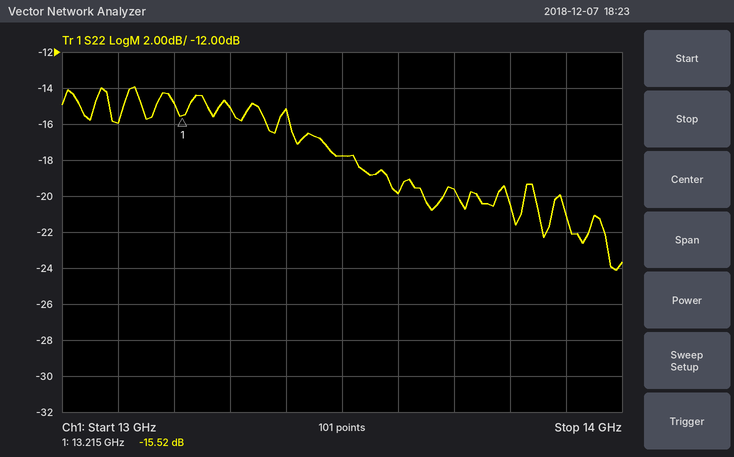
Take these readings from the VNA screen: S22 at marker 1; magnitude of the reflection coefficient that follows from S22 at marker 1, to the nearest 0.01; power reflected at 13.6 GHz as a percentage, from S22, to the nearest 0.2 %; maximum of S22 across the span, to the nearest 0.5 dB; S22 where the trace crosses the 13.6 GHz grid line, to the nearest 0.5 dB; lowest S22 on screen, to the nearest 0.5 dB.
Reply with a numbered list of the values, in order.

1. -15.52 dB
2. 0.17
3. 1.0 %
4. -14.0 dB
5. -20.0 dB
6. -24.0 dB
